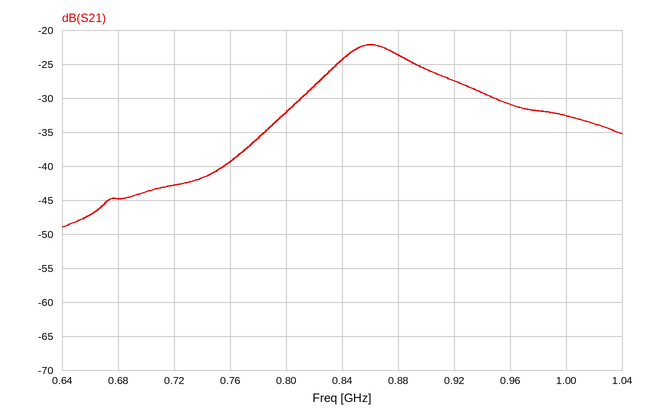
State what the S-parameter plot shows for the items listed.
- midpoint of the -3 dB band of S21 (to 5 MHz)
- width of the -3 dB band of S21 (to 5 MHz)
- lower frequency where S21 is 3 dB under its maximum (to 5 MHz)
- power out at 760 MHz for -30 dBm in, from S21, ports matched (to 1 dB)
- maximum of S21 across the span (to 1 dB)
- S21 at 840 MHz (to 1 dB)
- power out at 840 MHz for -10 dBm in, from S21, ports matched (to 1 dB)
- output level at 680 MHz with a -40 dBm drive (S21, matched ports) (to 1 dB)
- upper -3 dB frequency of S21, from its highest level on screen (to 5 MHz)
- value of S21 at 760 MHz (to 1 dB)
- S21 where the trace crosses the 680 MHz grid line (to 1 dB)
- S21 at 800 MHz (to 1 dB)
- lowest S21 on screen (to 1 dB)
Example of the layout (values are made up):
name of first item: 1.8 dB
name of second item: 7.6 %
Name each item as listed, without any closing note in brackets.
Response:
midpoint of the -3 dB band of S21: 865 MHz
width of the -3 dB band of S21: 60 MHz
lower frequency where S21 is 3 dB under its maximum: 835 MHz
power out at 760 MHz for -30 dBm in, from S21, ports matched: -69 dBm
maximum of S21 across the span: -22 dB
S21 at 840 MHz: -24 dB
power out at 840 MHz for -10 dBm in, from S21, ports matched: -34 dBm
output level at 680 MHz with a -40 dBm drive (S21, matched ports): -85 dBm
upper -3 dB frequency of S21, from its highest level on screen: 895 MHz
value of S21 at 760 MHz: -39 dB
S21 where the trace crosses the 680 MHz grid line: -45 dB
S21 at 800 MHz: -32 dB
lowest S21 on screen: -49 dB
